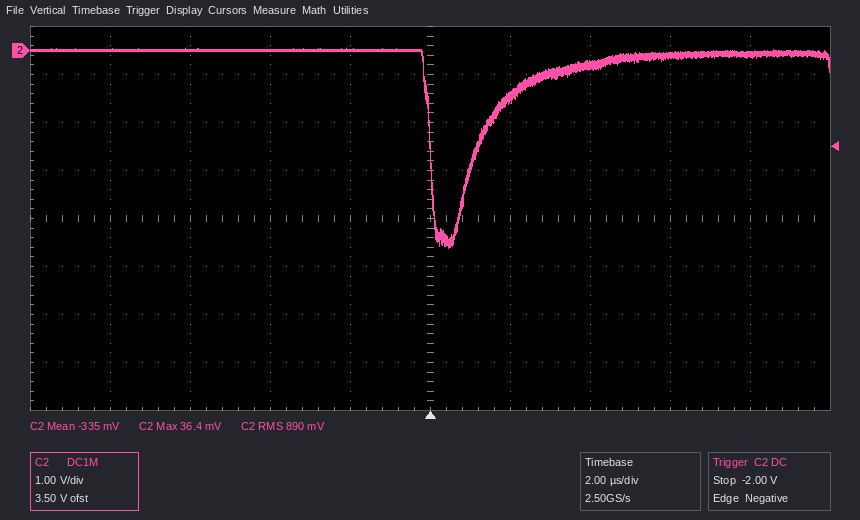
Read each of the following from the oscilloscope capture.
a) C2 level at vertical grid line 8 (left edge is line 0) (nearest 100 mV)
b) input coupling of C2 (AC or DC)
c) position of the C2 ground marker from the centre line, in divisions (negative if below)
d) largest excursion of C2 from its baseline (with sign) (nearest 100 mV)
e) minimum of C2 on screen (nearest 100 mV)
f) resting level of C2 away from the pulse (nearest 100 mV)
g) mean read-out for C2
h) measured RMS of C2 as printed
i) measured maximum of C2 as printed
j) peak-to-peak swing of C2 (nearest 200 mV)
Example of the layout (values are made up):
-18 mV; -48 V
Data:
-100 mV; DC; +3.5 div; -4.1 V; -4.1 V; 0.0 V; -335 mV; 890 mV; 36.4 mV; 4.2 V
